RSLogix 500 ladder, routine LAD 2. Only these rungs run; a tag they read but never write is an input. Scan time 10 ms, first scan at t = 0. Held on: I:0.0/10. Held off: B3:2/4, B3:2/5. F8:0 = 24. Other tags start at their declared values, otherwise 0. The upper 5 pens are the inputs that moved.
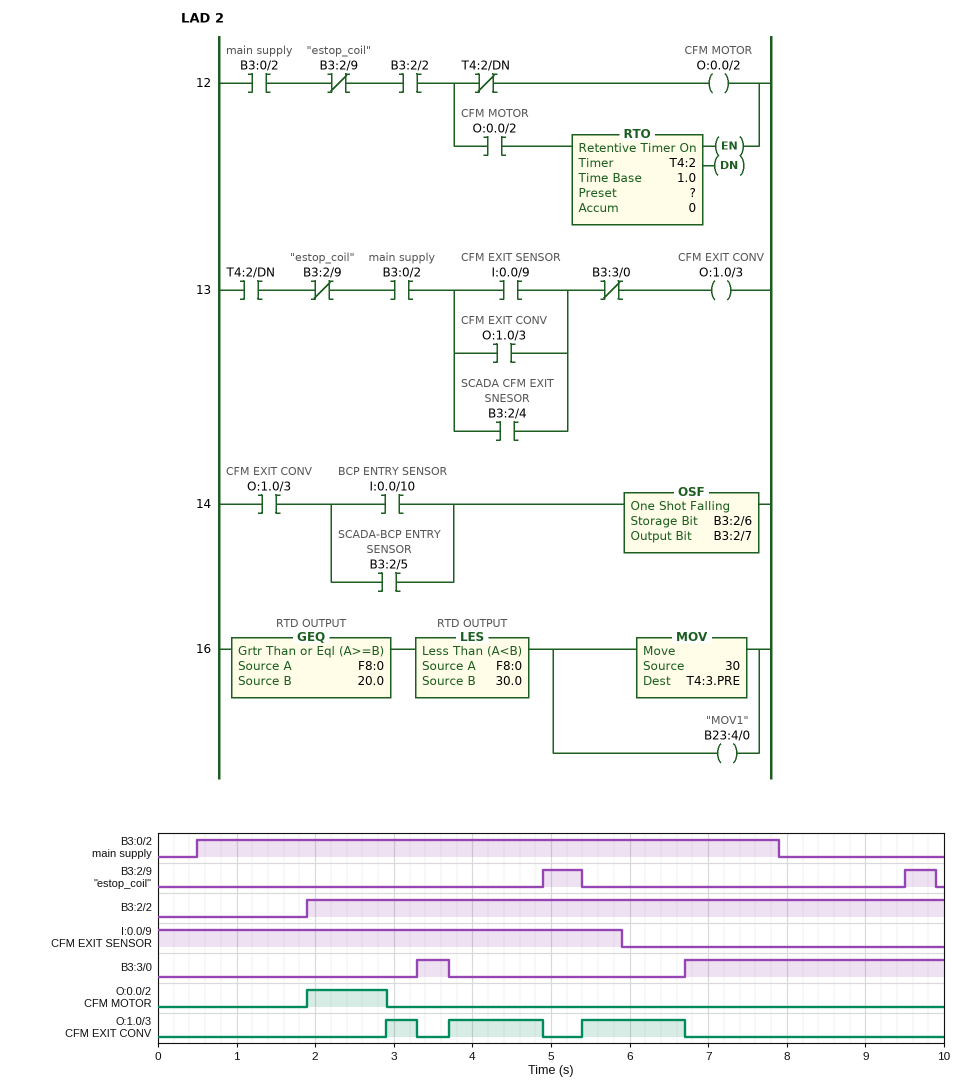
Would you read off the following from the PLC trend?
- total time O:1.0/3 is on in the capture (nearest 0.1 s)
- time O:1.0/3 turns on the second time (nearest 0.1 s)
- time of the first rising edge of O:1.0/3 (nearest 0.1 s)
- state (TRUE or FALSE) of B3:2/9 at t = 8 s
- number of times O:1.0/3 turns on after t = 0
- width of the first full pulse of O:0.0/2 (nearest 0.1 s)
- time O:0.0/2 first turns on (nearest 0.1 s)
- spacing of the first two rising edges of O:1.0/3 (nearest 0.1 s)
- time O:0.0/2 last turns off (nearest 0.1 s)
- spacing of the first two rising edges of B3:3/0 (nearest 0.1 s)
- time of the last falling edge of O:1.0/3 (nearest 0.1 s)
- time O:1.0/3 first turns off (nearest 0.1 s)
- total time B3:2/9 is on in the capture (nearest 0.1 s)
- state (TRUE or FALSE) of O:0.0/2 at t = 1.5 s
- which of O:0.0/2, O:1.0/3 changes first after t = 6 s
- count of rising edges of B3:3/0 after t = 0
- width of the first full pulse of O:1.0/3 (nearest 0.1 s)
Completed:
2.9 s
3.7 s
2.9 s
FALSE
3
1.0 s
1.9 s
0.8 s
2.9 s
3.4 s
6.7 s
3.3 s
0.9 s
FALSE
O:1.0/3
2
0.4 s
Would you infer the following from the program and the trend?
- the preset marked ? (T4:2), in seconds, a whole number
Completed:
1 s
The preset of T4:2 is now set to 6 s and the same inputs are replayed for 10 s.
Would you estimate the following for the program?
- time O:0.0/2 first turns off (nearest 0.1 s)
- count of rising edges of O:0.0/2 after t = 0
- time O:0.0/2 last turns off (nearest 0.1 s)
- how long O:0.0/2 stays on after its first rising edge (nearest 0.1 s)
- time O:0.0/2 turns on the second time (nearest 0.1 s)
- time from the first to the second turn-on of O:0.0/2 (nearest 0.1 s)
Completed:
4.9 s
2
7.9 s
3.0 s
5.4 s
3.5 s
